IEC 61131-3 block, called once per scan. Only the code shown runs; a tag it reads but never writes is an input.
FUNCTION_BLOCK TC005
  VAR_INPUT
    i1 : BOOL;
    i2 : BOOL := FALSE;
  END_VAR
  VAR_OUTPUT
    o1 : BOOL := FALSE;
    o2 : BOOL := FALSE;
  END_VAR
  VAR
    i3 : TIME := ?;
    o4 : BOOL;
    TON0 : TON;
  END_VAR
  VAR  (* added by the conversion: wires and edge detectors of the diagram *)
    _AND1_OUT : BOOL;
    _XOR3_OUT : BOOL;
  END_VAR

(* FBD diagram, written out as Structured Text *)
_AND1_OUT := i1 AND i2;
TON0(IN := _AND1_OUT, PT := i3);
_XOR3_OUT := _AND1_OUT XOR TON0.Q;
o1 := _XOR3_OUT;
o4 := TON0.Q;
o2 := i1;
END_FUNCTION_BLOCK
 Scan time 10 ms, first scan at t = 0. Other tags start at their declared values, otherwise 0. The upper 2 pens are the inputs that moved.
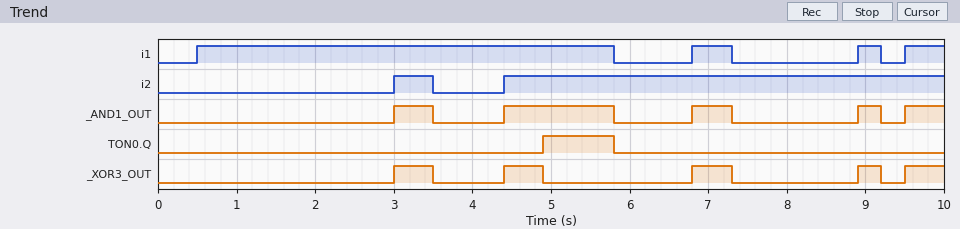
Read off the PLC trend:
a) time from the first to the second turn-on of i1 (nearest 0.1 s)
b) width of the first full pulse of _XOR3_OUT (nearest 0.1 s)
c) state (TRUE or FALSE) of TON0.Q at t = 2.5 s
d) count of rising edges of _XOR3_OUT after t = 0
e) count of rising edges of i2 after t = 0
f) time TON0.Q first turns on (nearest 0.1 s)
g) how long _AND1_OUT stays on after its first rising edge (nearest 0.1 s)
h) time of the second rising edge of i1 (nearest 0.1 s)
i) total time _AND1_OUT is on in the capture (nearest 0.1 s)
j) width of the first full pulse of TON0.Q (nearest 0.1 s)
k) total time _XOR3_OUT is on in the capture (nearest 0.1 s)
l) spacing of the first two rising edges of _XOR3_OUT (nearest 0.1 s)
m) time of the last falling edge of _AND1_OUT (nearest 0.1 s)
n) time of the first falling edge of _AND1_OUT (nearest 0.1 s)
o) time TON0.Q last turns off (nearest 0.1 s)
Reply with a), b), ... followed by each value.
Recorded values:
a) 6.3 s
b) 0.5 s
c) FALSE
d) 5
e) 2
f) 4.9 s
g) 0.5 s
h) 6.8 s
i) 3.2 s
j) 0.9 s
k) 2.3 s
l) 1.4 s
m) 9.2 s
n) 3.5 s
o) 5.8 s
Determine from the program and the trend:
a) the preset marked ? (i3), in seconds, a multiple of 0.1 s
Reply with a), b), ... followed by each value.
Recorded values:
a) 0.5 s
